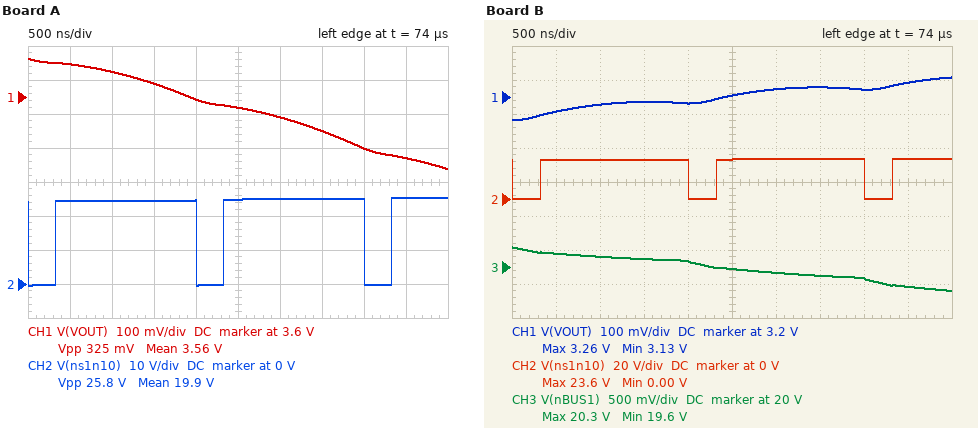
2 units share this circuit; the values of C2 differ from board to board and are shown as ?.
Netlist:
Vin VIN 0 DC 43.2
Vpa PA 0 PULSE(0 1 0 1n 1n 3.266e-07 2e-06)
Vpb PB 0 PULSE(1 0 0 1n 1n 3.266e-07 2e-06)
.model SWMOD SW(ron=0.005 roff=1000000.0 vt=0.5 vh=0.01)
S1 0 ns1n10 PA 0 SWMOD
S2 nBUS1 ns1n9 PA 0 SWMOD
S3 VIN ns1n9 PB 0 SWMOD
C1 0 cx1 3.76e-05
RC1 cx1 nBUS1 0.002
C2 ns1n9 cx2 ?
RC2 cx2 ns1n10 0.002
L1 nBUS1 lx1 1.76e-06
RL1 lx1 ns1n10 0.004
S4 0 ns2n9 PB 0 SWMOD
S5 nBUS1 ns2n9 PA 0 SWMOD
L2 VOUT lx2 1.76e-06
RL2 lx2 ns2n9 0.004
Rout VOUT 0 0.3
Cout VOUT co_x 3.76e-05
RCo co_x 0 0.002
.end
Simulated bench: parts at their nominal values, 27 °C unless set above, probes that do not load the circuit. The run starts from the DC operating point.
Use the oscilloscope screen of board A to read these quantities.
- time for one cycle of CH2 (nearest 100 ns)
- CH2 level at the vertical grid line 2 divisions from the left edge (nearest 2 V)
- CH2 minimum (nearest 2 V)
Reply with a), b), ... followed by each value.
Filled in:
a) 2.0 µs
b) 24 V
c) 0 V
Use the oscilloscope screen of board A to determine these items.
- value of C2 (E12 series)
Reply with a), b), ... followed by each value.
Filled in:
a) 120 µF
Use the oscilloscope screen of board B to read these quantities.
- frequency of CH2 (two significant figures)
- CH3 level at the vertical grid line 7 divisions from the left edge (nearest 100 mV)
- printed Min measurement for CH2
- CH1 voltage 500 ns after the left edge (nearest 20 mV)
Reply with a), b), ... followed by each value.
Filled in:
a) 500 kHz
b) 19.9 V
c) 0.00 V
d) 3.16 V
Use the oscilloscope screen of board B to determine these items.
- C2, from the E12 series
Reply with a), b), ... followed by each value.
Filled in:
a) 27 µF
